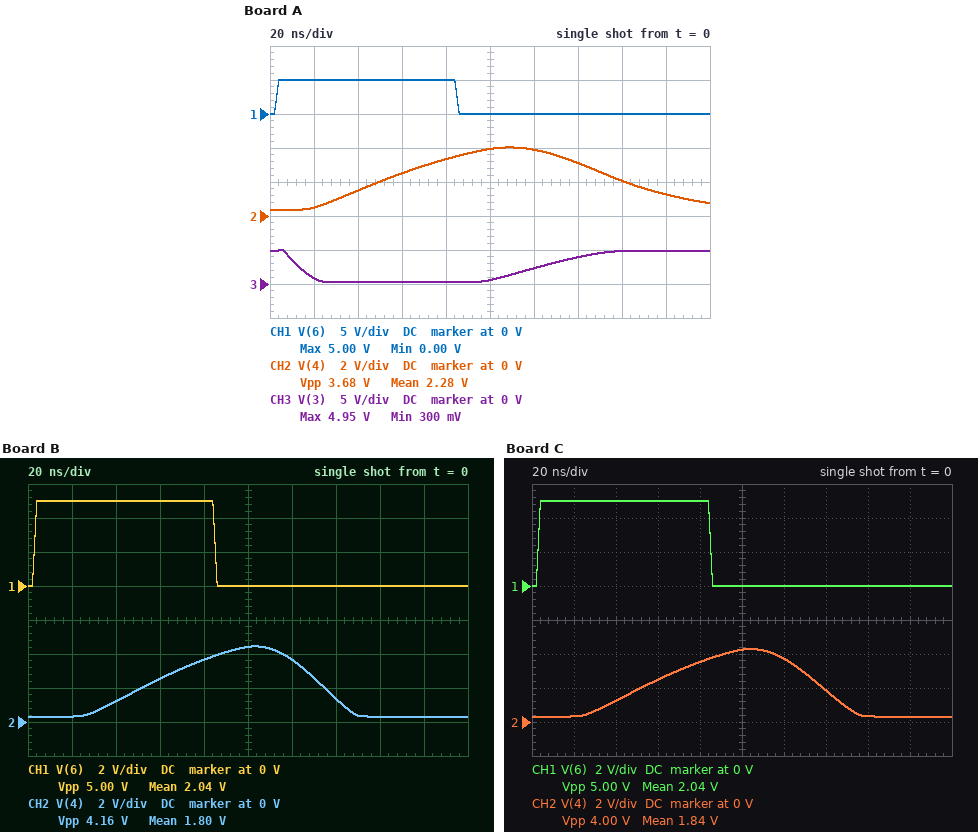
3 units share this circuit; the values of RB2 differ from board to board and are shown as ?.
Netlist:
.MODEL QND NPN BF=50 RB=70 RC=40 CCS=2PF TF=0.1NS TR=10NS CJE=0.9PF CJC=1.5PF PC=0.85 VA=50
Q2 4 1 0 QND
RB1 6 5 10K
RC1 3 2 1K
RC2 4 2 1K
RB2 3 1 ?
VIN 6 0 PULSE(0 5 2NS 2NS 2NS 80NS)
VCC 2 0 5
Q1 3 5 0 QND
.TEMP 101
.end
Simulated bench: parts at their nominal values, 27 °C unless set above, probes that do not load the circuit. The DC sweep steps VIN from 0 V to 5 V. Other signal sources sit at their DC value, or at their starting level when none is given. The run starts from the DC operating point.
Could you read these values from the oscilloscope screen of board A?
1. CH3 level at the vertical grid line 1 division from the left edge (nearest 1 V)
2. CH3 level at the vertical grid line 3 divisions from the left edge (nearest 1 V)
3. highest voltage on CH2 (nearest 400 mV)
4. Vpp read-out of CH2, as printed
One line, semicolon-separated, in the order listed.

1 V; 0 V; 4.0 V; 3.68 V
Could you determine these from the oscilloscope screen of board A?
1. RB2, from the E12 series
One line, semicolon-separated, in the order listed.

33 kΩ
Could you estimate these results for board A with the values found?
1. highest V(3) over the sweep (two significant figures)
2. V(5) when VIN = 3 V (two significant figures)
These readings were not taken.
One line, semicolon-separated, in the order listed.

4.9 V; 740 mV
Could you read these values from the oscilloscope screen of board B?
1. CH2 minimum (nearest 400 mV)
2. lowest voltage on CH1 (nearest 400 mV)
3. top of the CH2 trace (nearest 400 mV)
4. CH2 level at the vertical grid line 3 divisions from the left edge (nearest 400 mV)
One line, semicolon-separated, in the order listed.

400 mV; 0 V; 4.4 V; 2.4 V
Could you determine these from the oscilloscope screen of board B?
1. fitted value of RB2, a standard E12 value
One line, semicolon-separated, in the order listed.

12 kΩ
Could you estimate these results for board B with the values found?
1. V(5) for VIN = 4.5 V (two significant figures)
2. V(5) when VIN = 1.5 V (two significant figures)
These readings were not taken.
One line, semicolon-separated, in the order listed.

750 mV; 720 mV
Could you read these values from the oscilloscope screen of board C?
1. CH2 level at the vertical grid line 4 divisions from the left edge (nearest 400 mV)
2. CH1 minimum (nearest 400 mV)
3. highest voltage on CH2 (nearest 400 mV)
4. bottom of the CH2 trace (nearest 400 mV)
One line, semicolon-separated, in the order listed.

3.6 V; 0 V; 4.4 V; 400 mV
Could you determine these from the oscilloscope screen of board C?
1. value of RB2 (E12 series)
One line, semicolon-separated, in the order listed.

15 kΩ
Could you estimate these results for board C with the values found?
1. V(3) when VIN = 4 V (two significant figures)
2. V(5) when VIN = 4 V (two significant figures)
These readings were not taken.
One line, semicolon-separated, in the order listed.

290 mV; 750 mV
